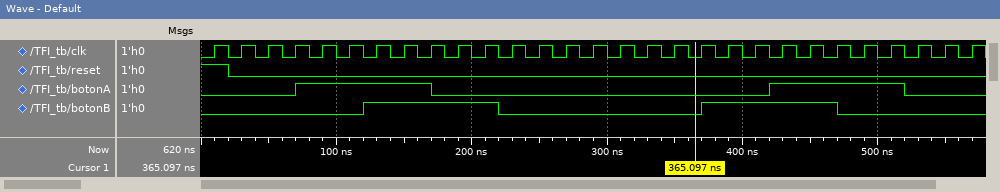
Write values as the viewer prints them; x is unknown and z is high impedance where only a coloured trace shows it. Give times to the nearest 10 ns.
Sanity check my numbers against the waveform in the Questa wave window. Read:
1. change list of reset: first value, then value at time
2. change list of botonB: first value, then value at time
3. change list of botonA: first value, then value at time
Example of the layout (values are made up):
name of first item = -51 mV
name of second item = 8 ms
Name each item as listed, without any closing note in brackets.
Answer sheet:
change list of reset: first value, then value at time = 1, 0 at 20 ns
change list of botonB: first value, then value at time = 0, 1 at 120 ns, 0 at 220 ns, 1 at 370 ns, 0 at 470 ns
change list of botonA: first value, then value at time = 0, 1 at 70 ns, 0 at 170 ns, 1 at 420 ns, 0 at 520 ns
